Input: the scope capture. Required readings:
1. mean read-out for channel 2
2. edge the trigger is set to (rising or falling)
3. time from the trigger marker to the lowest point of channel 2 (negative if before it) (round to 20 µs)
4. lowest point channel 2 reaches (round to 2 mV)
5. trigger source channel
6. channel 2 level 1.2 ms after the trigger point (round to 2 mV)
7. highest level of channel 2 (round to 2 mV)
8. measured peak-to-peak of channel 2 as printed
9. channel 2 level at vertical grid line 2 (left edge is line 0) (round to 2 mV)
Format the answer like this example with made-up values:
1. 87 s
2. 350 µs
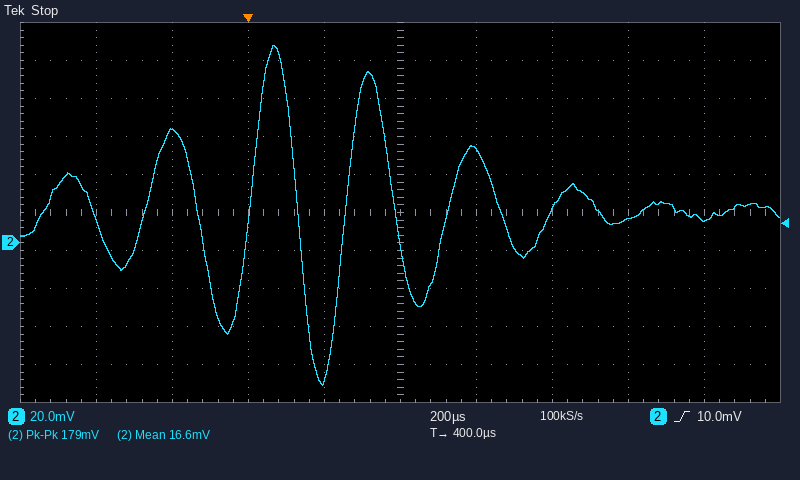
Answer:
1. 16.6 mV
2. rising
3. +200 µs
4. -76 mV
5. channel 2
6. 12 mV
7. 104 mV
8. 179 mV
9. 58 mV
